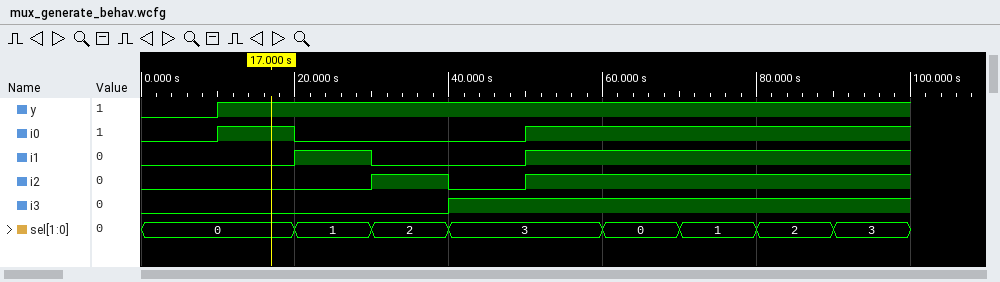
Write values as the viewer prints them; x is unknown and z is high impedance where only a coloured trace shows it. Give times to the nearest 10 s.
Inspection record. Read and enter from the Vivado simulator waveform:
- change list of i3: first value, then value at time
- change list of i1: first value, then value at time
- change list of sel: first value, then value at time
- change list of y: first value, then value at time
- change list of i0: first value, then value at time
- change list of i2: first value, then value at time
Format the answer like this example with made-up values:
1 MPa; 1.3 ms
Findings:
0, 1 at 40 s; 0, 1 at 20 s, 0 at 30 s, 1 at 50 s; 0, 1 at 20 s, 2 at 30 s, 3 at 40 s, 0 at 60 s, 1 at 70 s, 2 at 80 s, 3 at 90 s; 0, 1 at 10 s; 0, 1 at 10 s, 0 at 20 s, 1 at 50 s; 0, 1 at 30 s, 0 at 40 s, 1 at 50 s
